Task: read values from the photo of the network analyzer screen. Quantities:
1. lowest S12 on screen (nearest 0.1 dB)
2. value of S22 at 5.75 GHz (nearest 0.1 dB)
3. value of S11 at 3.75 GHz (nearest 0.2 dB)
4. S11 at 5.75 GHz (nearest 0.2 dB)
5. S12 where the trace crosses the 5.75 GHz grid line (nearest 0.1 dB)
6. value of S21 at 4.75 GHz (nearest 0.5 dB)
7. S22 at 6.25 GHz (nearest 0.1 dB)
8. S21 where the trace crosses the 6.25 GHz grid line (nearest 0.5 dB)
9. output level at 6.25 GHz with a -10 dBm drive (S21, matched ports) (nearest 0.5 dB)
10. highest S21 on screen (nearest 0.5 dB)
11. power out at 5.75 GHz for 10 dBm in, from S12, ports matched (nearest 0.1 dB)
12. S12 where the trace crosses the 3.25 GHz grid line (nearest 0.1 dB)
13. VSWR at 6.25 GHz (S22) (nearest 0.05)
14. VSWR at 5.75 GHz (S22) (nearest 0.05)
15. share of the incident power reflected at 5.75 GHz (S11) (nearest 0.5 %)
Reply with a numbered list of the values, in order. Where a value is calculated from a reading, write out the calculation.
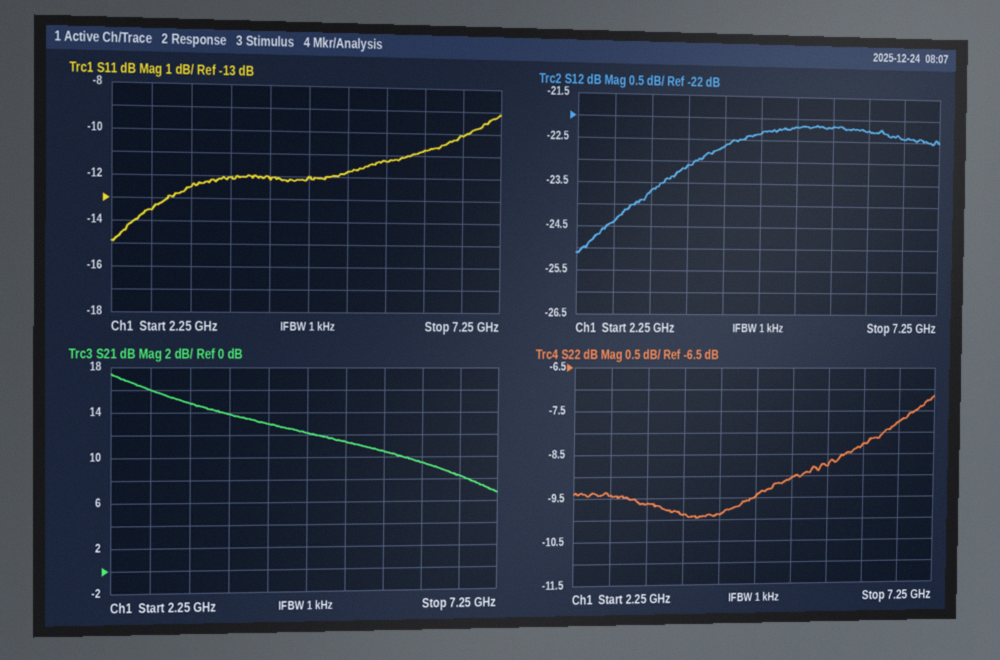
1. -25.1 dB
2. -8.8 dB
3. -12.0 dB
4. -11.2 dB
5. -22.2 dB
6. 12.0 dB
7. -8.3 dB
8. 9.5 dB
9. -10 dBm + (9.5 dB) = -0.5 dBm
10. 17.5 dB
11. 10 dBm + (-22.2 dB) = -12.2 dBm
12. -23.7 dB
13. |Γ| = 10^(-8.3/20) = 0.3846; VSWR = (1 + 0.3846)/(1 − 0.3846) ≈ 2.25
14. |Γ| = 10^(-8.8/20) = 0.3631; VSWR = (1 + 0.3631)/(1 − 0.3631) ≈ 2.14, so 2.15 to the nearest 0.05
15. 10^(-11.2/10) ≈ 7.59 %, so 7.5 % to the nearest 0.5 %
